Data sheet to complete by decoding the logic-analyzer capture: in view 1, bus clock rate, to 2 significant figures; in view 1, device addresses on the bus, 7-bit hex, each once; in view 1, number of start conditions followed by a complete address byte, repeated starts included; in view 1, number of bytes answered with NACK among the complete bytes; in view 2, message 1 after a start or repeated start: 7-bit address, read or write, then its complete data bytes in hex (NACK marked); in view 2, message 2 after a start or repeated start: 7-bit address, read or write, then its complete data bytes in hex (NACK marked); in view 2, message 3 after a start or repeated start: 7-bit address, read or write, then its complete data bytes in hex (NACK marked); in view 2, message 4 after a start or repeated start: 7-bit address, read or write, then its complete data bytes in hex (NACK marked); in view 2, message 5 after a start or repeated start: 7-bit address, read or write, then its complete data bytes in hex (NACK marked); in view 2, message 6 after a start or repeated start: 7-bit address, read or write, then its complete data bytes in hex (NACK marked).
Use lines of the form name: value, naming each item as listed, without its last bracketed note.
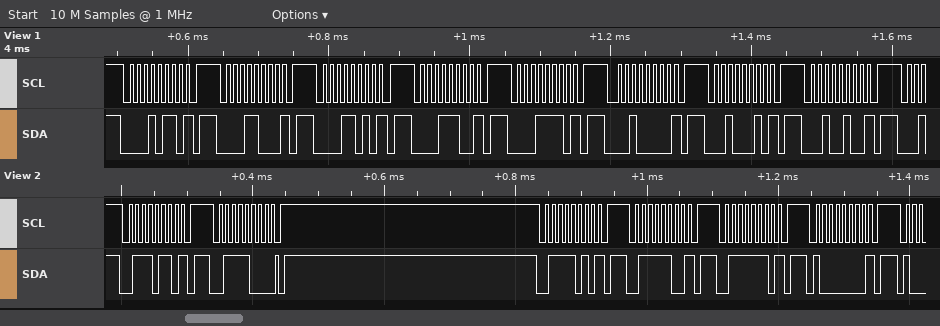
in view 1, bus clock rate, to 2 significant figures: 100 kHz
in view 1, device addresses on the bus, 7-bit hex, each once: 0x0B 0x0C 0x0D 0x0E 0x0F 0x10 0x11 0x12
in view 1, number of start conditions followed by a complete address byte, repeated starts included: 8
in view 1, number of bytes answered with NACK among the complete bytes: 8
in view 2, message 1 after a start or repeated start: 7-bit address, read or write, then its complete data bytes in hex: 0x3B write NACK
in view 2, message 2 after a start or repeated start: 7-bit address, read or write, then its complete data bytes in hex: 0x3C write
in view 2, message 3 after a start or repeated start: 7-bit address, read or write, then its complete data bytes in hex: 0x3D write NACK
in view 2, message 4 after a start or repeated start: 7-bit address, read or write, then its complete data bytes in hex: 0x3E write NACK
in view 2, message 5 after a start or repeated start: 7-bit address, read or write, then its complete data bytes in hex: 0x3F write NACK
in view 2, message 6 after a start or repeated start: 7-bit address, read or write, then its complete data bytes in hex: 0x40 write NACK
